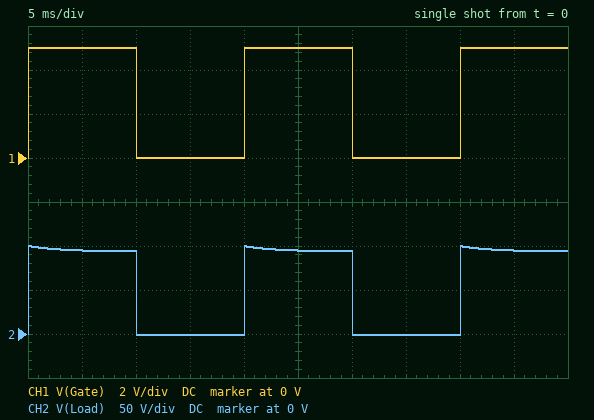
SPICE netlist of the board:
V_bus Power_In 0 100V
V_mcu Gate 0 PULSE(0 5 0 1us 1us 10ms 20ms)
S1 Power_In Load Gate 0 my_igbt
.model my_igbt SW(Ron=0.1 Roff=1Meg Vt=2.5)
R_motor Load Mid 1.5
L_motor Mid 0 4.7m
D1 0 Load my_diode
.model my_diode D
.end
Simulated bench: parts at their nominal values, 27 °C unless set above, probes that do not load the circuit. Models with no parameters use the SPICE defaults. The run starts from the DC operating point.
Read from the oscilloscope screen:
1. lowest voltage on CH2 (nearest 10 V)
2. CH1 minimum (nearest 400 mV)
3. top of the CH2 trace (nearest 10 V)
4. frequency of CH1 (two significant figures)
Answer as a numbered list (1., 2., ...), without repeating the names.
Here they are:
1. 0 V
2. 0 V
3. 100 V
4. 50 Hz
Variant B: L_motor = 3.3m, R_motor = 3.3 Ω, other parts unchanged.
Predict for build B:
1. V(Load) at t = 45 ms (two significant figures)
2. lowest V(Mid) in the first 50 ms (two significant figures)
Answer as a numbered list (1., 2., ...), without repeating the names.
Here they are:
1. 97 V
2. -98 V
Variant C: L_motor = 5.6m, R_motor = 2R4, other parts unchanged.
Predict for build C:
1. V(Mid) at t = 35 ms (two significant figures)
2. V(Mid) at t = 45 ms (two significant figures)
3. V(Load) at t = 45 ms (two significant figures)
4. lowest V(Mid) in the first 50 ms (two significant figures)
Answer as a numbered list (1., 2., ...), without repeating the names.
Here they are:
1. -11 V
2. 11 V
3. 96 V
4. -96 V
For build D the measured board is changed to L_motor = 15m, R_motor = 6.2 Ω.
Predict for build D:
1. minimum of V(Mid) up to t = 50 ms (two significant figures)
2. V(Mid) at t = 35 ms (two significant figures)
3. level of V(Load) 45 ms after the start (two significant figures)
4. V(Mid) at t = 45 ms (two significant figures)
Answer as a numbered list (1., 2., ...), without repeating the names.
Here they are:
1. -98 V
2. -12 V
3. 99 V
4. 12 V
